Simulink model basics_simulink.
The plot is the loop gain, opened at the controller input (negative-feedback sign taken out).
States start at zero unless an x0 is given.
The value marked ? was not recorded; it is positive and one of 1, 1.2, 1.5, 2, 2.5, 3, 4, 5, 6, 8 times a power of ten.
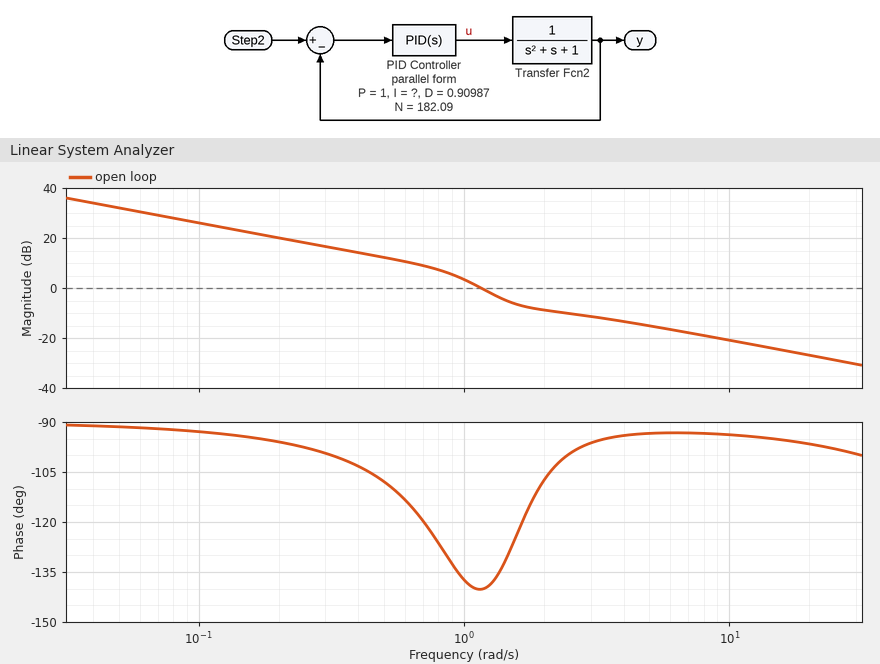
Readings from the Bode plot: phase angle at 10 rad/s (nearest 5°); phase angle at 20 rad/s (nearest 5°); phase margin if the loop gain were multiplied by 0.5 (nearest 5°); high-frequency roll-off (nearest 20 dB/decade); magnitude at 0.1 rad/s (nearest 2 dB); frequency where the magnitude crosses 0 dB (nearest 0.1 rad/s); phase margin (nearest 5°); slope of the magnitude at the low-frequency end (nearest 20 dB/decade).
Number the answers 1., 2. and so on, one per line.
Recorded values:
1. -95°
2. -95°
3. 50°
4. -20 dB/decade
5. 26 dB
6. 1.2 rad/s
7. 40°
8. -20 dB/decade
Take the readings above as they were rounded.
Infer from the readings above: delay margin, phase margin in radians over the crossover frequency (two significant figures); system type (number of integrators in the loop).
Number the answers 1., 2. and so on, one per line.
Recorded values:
1. 0.58 s
2. 1
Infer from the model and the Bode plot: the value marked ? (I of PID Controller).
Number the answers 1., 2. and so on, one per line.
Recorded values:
1. 2
